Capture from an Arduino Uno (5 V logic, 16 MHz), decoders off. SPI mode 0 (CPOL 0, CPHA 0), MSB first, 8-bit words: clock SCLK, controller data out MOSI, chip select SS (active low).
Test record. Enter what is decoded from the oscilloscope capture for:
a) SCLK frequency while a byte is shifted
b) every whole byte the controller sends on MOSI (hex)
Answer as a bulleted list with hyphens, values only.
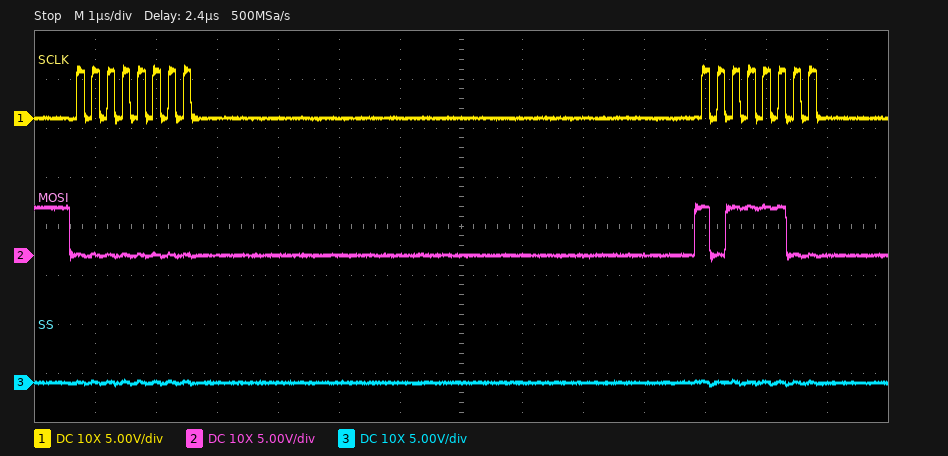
- 4 MHz
- 00 BC
